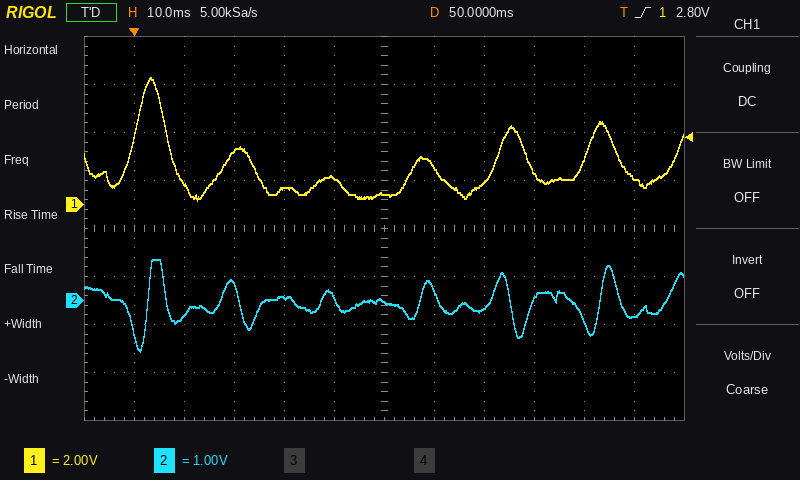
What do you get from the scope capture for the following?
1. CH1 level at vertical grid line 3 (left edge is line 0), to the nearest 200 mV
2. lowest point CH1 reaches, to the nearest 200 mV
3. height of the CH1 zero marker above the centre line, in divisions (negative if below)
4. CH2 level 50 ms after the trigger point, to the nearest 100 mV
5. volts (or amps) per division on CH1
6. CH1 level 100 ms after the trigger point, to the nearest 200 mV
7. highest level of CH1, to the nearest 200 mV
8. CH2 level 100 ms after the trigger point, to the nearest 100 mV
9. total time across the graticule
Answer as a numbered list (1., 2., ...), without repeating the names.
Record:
1. 2.2 V
2. 200 mV
3. +0.5 div
4. 0.0 V
5. 2 V
6. 1.2 V
7. 5.2 V
8. -300 mV
9. 120 ms
